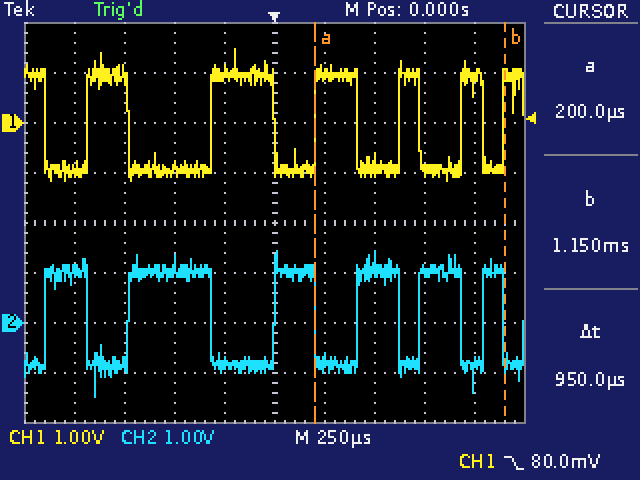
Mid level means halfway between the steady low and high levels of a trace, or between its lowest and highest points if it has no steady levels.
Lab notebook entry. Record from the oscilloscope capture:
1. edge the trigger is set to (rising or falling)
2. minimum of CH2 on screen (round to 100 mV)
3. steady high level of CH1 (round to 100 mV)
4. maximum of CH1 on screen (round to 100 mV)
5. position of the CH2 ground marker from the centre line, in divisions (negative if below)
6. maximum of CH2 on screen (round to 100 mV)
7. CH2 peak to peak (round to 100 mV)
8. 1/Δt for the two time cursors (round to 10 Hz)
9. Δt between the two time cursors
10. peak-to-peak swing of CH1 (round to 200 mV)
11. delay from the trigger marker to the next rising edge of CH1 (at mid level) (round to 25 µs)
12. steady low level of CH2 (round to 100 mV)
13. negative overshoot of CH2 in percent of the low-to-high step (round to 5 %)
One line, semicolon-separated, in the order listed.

falling; -1.5 V; 1.0 V; 1.5 V; -2.0 div; 1.4 V; 2.9 V; 1.05 kHz; 950 µs; 2.6 V; 200 µs; -800 mV; 35 %
